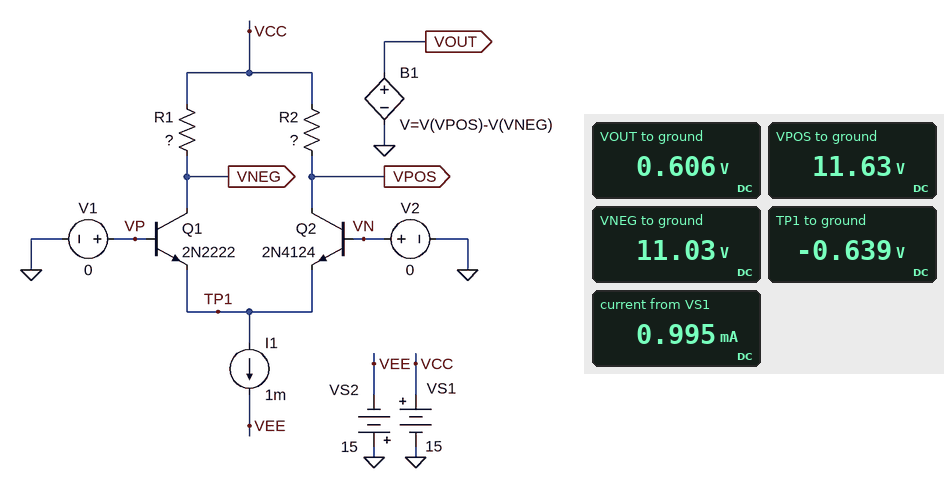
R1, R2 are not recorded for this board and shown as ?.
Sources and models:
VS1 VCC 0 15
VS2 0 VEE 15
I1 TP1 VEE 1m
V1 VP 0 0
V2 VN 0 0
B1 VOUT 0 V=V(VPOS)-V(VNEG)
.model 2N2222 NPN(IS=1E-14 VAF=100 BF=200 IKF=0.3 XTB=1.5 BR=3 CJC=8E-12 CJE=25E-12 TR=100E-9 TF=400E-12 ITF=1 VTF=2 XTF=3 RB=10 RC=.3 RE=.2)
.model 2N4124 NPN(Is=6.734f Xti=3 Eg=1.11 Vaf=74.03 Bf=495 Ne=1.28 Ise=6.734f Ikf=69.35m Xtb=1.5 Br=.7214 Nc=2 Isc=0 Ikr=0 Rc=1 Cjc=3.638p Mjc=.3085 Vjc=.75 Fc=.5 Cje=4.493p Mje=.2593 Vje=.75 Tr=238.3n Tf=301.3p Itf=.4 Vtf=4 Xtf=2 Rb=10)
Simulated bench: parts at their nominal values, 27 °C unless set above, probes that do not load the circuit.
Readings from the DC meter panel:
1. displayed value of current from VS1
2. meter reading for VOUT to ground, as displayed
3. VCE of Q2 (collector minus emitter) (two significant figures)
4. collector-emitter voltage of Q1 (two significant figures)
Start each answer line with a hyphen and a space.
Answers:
- 0.995 mA
- 0.606 V
- 12 V
- 12 V
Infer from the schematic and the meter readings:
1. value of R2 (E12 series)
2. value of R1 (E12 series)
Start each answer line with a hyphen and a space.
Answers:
- 8.2 kΩ
- 6.8 kΩ
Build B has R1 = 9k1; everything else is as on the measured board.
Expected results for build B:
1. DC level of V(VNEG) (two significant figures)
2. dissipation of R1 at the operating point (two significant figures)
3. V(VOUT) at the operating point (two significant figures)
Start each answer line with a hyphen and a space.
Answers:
- 9.7 V
- 3.1 mW
- 1.9 V
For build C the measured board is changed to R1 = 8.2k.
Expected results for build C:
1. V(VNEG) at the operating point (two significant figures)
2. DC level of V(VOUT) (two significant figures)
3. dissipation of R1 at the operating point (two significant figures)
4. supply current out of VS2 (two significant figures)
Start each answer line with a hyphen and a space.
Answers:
- 10 V
- 1.4 V
- 2.8 mW
- 1.0 mA
